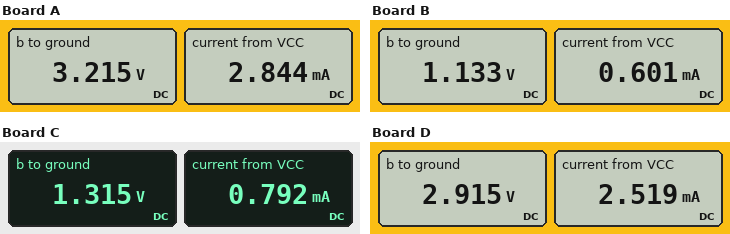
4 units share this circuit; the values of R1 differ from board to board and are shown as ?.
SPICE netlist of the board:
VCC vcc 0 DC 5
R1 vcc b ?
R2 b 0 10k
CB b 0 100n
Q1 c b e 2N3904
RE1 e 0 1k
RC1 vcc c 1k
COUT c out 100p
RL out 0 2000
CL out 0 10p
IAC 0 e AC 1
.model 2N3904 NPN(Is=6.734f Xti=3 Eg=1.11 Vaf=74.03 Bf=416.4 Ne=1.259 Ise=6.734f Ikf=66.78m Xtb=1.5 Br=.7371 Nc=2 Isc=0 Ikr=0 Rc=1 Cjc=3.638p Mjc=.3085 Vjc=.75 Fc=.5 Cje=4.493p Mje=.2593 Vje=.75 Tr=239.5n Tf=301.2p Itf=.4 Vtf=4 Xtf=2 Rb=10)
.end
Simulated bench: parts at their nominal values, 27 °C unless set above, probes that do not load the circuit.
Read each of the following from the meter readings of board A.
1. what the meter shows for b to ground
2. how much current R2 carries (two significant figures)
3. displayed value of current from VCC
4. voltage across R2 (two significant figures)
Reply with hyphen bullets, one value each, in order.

- 3.215 V
- 320 µA
- 2.844 mA
- 3.2 V
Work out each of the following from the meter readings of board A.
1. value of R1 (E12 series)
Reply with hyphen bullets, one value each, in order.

- 3.9 kΩ
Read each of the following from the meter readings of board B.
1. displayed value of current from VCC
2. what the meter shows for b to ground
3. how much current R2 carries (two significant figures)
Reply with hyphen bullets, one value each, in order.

- 0.601 mA
- 1.133 V
- 110 µA
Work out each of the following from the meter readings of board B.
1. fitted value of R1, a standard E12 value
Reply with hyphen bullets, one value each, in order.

- 33 kΩ
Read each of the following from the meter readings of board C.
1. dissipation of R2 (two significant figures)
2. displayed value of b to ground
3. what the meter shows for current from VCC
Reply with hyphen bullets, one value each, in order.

- 170 µW
- 1.315 V
- 0.792 mA
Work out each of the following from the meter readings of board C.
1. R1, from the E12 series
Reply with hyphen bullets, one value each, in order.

- 27 kΩ
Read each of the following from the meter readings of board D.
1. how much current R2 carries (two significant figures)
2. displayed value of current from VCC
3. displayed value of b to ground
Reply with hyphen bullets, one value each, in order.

- 290 µA
- 2.519 mA
- 2.915 V
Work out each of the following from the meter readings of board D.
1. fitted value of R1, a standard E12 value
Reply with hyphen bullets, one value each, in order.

- 6.8 kΩ
